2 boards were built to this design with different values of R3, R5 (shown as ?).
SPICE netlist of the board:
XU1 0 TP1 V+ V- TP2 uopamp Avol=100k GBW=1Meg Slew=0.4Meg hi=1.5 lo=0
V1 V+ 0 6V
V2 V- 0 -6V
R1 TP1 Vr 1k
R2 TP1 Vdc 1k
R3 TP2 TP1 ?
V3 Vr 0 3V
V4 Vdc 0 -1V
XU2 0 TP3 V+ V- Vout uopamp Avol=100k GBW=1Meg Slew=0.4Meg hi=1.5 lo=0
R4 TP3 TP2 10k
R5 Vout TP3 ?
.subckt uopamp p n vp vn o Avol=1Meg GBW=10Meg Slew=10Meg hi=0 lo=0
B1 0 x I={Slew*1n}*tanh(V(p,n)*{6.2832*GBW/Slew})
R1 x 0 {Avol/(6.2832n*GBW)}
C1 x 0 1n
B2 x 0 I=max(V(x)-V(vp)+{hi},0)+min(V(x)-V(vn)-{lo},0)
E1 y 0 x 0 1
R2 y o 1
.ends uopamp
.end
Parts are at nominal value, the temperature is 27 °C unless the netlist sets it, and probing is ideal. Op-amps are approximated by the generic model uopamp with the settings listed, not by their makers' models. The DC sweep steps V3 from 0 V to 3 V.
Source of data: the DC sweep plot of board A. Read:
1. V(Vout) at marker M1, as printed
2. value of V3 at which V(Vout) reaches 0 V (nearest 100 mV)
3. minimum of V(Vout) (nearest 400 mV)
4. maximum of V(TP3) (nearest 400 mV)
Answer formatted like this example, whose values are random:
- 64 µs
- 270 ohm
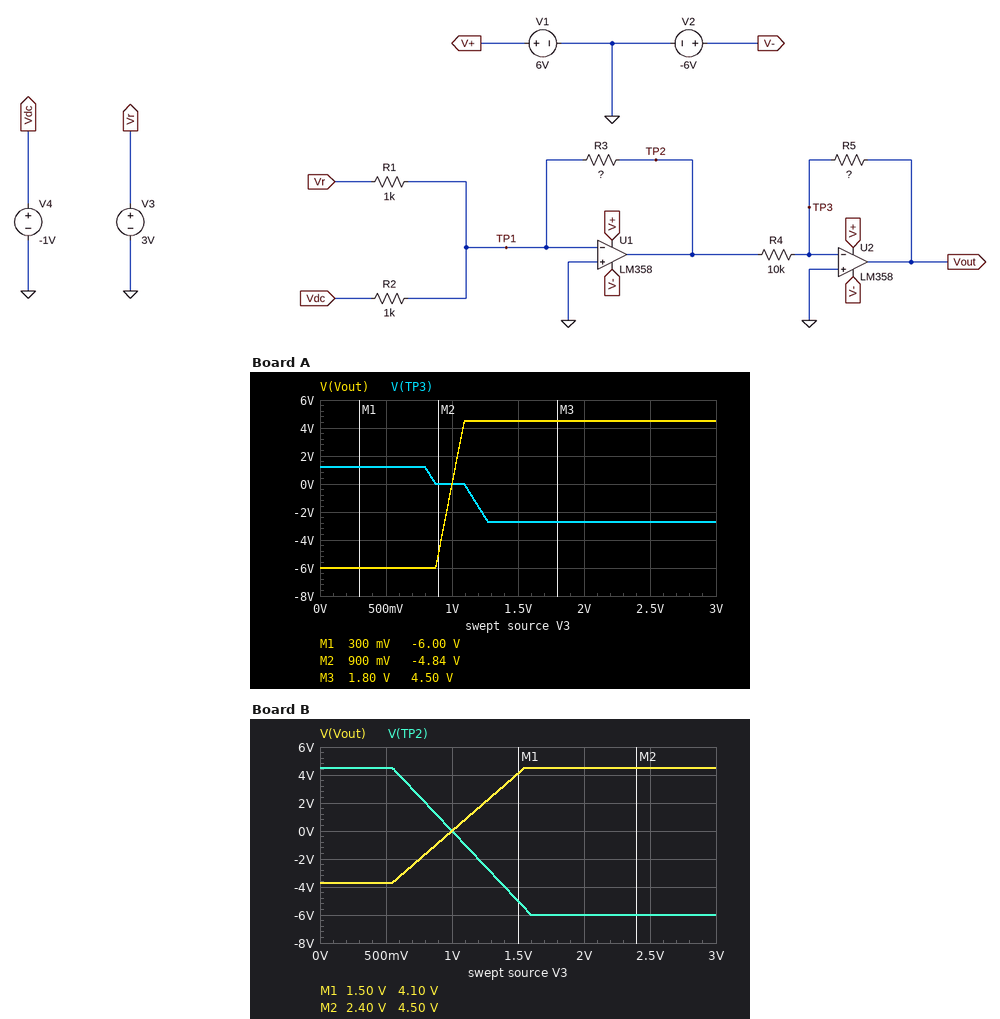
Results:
- -6.00 V
- 1.0 V
- -6.0 V
- 1.2 V
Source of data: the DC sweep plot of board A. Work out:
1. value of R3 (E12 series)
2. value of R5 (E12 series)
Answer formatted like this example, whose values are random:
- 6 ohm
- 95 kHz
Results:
- 22 kΩ
- 22 kΩ
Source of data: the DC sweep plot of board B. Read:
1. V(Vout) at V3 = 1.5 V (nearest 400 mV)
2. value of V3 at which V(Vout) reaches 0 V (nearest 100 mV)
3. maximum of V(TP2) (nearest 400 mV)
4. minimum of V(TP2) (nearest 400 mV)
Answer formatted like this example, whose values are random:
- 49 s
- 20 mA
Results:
- 4.0 V
- 1.0 V
- 4.4 V
- -6.0 V
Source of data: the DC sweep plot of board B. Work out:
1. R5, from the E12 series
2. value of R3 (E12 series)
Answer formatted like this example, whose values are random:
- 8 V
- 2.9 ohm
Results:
- 8.2 kΩ
- 10 kΩ
